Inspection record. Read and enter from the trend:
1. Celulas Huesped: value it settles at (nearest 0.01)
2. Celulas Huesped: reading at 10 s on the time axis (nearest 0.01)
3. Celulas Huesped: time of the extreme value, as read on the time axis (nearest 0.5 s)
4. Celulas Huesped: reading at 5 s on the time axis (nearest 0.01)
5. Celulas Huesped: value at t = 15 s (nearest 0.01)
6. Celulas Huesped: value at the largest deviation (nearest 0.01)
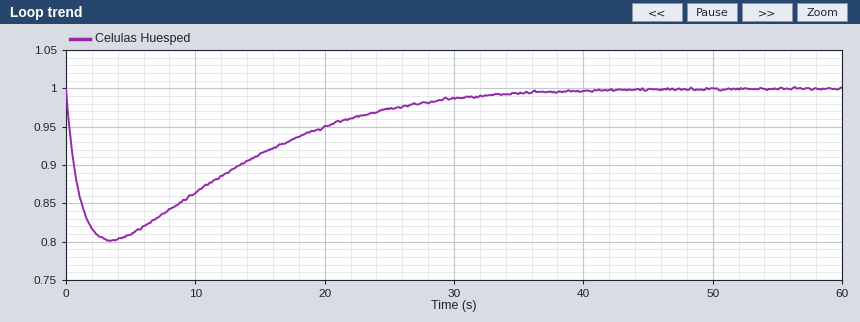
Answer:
1.00
0.86
3.5 s
0.81
0.91
0.80
